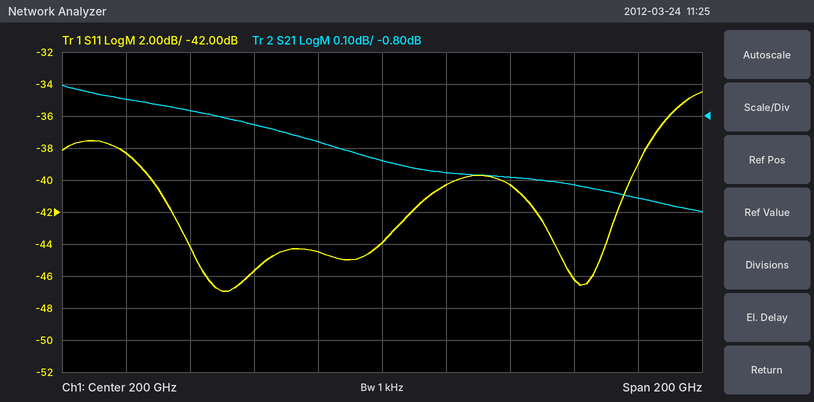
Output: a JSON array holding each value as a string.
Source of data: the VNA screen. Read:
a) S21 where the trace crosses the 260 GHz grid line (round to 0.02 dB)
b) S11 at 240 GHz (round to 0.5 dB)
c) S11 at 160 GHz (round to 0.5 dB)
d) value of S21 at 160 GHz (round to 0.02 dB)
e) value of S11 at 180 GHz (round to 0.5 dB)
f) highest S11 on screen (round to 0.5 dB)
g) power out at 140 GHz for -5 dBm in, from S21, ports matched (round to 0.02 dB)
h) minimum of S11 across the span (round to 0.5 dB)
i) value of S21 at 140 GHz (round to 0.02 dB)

["-1.02 dB", "-40.5 dB", "-45.5 dB", "-0.82 dB", "-44.5 dB", "-34.5 dB", "-5.78 dBm", "-47.0 dB", "-0.78 dB"]
